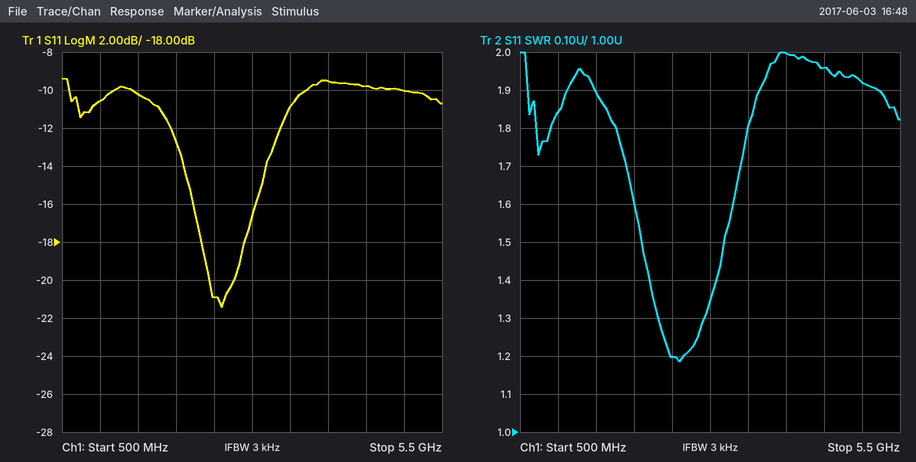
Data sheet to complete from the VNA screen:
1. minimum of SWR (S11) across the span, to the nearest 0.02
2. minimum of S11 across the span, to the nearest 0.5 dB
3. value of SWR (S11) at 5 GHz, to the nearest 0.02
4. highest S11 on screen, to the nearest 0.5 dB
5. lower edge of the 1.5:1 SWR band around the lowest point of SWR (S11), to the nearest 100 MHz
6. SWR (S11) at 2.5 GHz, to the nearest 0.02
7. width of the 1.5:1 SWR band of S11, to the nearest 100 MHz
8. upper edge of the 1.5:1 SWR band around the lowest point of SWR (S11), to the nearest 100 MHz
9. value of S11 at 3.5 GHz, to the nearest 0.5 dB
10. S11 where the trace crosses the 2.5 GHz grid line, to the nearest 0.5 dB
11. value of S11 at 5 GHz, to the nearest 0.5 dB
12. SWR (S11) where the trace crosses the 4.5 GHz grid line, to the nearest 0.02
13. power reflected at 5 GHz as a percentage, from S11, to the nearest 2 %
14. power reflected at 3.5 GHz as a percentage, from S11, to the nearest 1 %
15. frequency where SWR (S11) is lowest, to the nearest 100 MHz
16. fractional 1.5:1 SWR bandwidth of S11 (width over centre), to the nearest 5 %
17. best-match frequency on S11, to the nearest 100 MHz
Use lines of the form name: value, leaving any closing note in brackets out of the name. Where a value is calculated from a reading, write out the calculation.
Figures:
minimum of SWR (S11) across the span, to the nearest 0.02: 1.18
minimum of S11 across the span, to the nearest 0.5 dB: -21.5 dB
value of SWR (S11) at 5 GHz, to the nearest 0.02: 1.92
highest S11 on screen, to the nearest 0.5 dB: -9.5 dB
lower edge of the 1.5:1 SWR band around the lowest point of SWR (S11), to the nearest 100 MHz: 2.1 GHz
SWR (S11) at 2.5 GHz, to the nearest 0.02: 1.20
width of the 1.5:1 SWR band of S11, to the nearest 100 MHz: 3.2 GHz − 2.1 GHz = 1.1 GHz
upper edge of the 1.5:1 SWR band around the lowest point of SWR (S11), to the nearest 100 MHz: 3.2 GHz
value of S11 at 3.5 GHz, to the nearest 0.5 dB: -11.0 dB
S11 where the trace crosses the 2.5 GHz grid line, to the nearest 0.5 dB: -21.0 dB
value of S11 at 5 GHz, to the nearest 0.5 dB: -10.0 dB
SWR (S11) where the trace crosses the 4.5 GHz grid line, to the nearest 0.02: 1.96
power reflected at 5 GHz as a percentage, from S11, to the nearest 2 %: 10^(-10/10) ≈ 10 %
power reflected at 3.5 GHz as a percentage, from S11, to the nearest 1 %: 10^(-11/10) ≈ 8 %
frequency where SWR (S11) is lowest, to the nearest 100 MHz: 2.6 GHz
fractional 1.5:1 SWR bandwidth of S11 (width over centre), to the nearest 5 %: 1.1 GHz / 2.65 GHz ≈ 41.5 %, so 40 % to the nearest 5 %
best-match frequency on S11, to the nearest 100 MHz: 2.6 GHz
